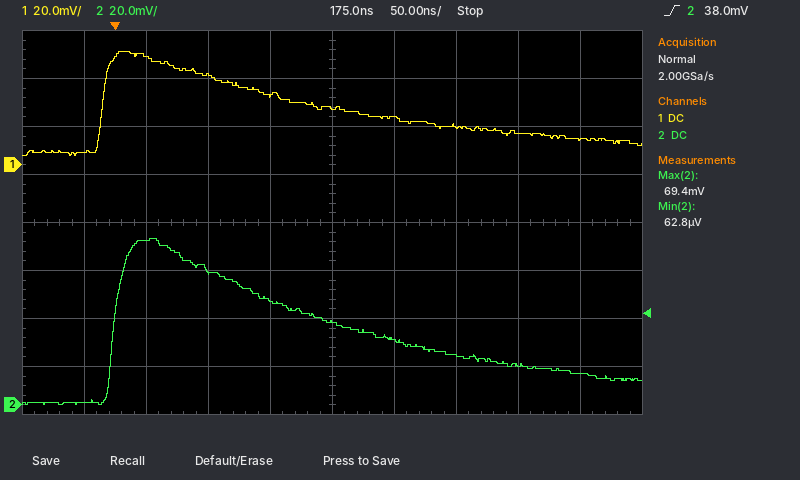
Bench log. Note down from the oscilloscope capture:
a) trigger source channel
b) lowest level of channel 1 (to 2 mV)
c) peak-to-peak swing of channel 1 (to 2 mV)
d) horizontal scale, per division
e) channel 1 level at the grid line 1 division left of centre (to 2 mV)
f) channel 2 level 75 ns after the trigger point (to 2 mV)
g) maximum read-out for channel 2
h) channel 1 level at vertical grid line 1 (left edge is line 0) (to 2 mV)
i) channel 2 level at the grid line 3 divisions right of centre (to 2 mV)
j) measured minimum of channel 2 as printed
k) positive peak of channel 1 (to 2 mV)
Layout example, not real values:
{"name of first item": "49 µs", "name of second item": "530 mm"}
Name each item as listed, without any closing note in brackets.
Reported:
{"trigger source channel": "channel 2", "lowest level of channel 1": "4 mV", "peak-to-peak swing of channel 1": "44 mV", "horizontal scale, per division": "50 ns", "channel 1 level at the grid line 1 division left of centre": "30 mV", "channel 2 level 75 ns after the trigger point": "56 mV", "maximum read-out for channel 2": "69.4 mV", "channel 1 level at vertical grid line 1 (left edge is line 0)": "6 mV", "channel 2 level at the grid line 3 divisions right of centre": "16 mV", "measured minimum of channel 2 as printed": "62.8 µV", "positive peak of channel 1": "48 mV"}
